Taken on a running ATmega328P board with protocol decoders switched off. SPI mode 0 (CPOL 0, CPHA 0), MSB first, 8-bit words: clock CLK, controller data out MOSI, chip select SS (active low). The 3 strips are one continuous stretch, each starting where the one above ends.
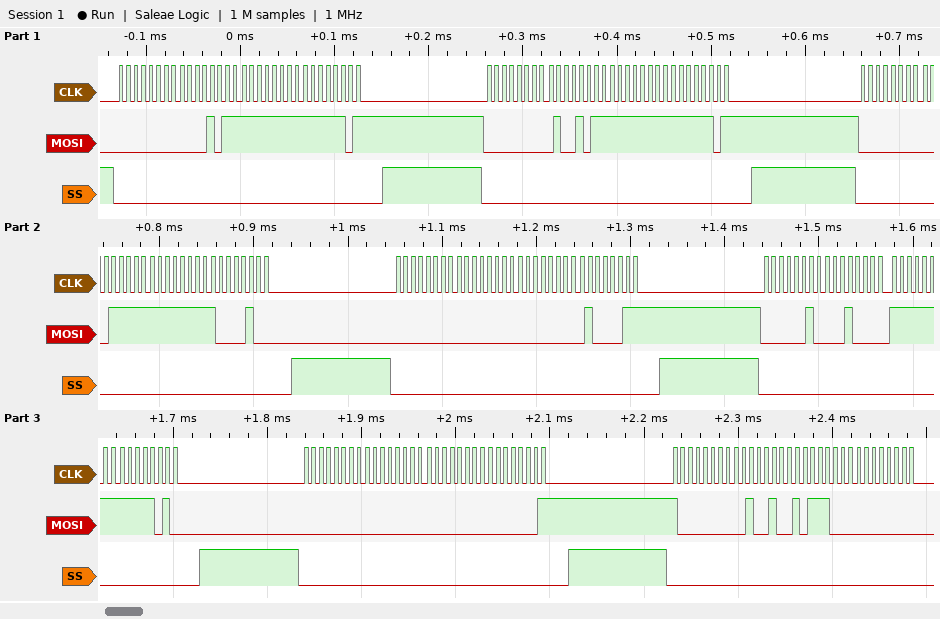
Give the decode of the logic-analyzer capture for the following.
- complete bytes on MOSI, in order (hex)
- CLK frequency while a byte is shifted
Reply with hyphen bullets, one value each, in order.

- 00 0B FF FD 00 4B FF FD 00 1F FF 84 00 00 00 43 02 10 FF FA 00 00 00 01 80 24 B8 00
- 125 kHz
